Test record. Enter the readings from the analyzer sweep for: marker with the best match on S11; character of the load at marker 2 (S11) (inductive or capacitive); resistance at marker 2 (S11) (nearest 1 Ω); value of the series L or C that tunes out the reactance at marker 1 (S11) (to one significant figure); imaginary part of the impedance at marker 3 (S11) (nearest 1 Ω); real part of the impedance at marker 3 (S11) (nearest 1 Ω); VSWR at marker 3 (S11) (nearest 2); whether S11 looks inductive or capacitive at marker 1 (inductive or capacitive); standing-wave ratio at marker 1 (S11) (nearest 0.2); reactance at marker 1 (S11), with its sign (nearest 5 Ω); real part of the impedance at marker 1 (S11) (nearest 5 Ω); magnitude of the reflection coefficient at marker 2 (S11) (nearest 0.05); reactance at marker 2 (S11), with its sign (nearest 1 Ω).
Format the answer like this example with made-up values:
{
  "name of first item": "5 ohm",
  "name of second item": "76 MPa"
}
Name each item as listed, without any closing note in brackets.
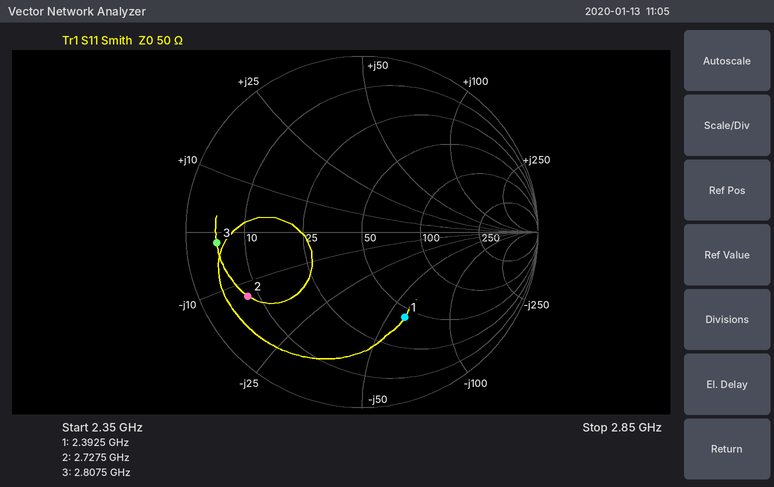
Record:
{
  "marker with the best match on S11": "marker 1",
  "character of the load at marker 2 (S11)": "capacitive",
  "resistance at marker 2 (S11)": "8 Ω",
  "value of the series L or C that tunes out the reactance at marker 1 (S11)": "4 nH",
  "imaginary part of the impedance at marker 3 (S11)": "-2 Ω",
  "real part of the impedance at marker 3 (S11)": "5 Ω",
  "VSWR at marker 3 (S11)": "10",
  "whether S11 looks inductive or capacitive at marker 1": "capacitive",
  "standing-wave ratio at marker 1 (S11)": "3.4",
  "reactance at marker 1 (S11), with its sign": "-60 Ω",
  "real part of the impedance at marker 1 (S11)": "45 Ω",
  "magnitude of the reflection coefficient at marker 2 (S11)": "0.75",
  "reactance at marker 2 (S11), with its sign": "-13 Ω"
}
